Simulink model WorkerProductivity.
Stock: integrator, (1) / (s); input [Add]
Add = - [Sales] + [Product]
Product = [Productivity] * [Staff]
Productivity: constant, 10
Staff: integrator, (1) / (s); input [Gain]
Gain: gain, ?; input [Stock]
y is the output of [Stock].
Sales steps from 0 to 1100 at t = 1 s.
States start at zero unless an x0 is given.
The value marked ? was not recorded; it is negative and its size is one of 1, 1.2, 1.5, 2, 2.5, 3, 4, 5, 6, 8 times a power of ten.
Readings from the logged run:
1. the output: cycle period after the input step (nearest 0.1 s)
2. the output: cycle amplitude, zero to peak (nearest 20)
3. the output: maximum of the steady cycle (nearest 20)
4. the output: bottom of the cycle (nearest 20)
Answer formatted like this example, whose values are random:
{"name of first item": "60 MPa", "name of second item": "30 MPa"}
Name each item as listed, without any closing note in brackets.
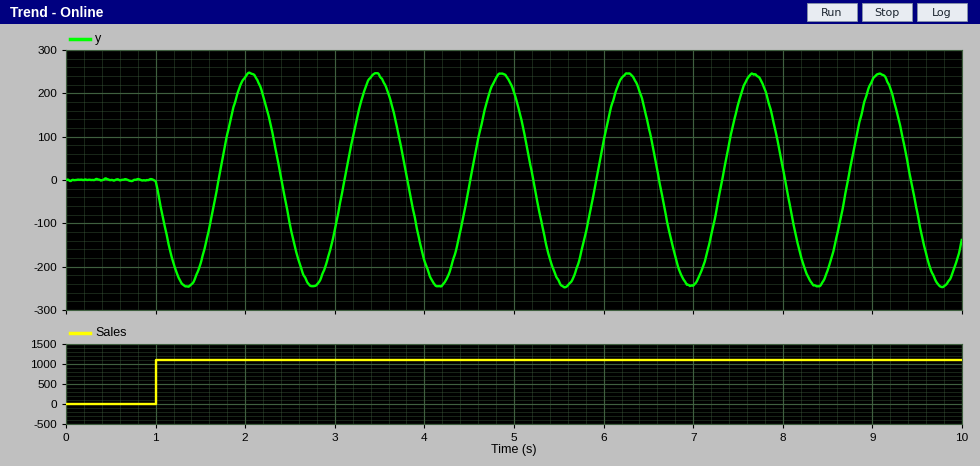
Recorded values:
{"the output: cycle period after the input step": "1.4 s", "the output: cycle amplitude, zero to peak": "240", "the output: maximum of the steady cycle": "240", "the output: bottom of the cycle": "-240"}
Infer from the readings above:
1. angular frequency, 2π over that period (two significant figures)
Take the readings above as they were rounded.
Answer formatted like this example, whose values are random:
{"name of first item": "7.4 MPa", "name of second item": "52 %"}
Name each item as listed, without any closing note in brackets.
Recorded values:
{"angular frequency, 2π over that period": "4.5 rad/s"}
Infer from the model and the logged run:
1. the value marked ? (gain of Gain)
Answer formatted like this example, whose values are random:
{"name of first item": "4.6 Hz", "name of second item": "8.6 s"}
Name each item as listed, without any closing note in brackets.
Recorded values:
{"the value marked ?": "-2"}
